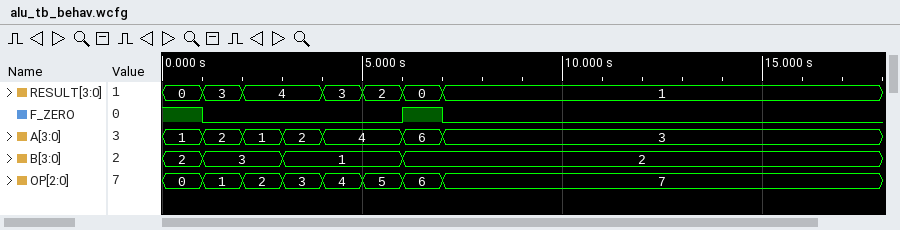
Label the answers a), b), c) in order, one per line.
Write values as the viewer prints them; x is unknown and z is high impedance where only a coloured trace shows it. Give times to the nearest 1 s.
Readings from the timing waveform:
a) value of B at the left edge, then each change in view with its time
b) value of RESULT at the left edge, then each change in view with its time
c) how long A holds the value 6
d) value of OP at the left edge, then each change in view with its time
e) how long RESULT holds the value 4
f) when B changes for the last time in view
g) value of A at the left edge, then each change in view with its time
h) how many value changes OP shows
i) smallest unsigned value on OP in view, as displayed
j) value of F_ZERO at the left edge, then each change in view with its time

a) 2, 3 at 1 s, 1 at 3 s, 2 at 6 s
b) 0, 3 at 1 s, 4 at 2 s, 3 at 4 s, 2 at 5 s, 0 at 6 s, 1 at 7 s
c) 1 s
d) 0, 1 at 1 s, 2 at 2 s, 3 at 3 s, 4 at 4 s, 5 at 5 s, 6 at 6 s, 7 at 7 s
e) 2 s
f) 6 s
g) 1, 2 at 1 s, 1 at 2 s, 2 at 3 s, 4 at 4 s, 6 at 6 s, 3 at 7 s
h) 7
i) 0
j) 1, 0 at 1 s, 1 at 6 s, 0 at 7 s
